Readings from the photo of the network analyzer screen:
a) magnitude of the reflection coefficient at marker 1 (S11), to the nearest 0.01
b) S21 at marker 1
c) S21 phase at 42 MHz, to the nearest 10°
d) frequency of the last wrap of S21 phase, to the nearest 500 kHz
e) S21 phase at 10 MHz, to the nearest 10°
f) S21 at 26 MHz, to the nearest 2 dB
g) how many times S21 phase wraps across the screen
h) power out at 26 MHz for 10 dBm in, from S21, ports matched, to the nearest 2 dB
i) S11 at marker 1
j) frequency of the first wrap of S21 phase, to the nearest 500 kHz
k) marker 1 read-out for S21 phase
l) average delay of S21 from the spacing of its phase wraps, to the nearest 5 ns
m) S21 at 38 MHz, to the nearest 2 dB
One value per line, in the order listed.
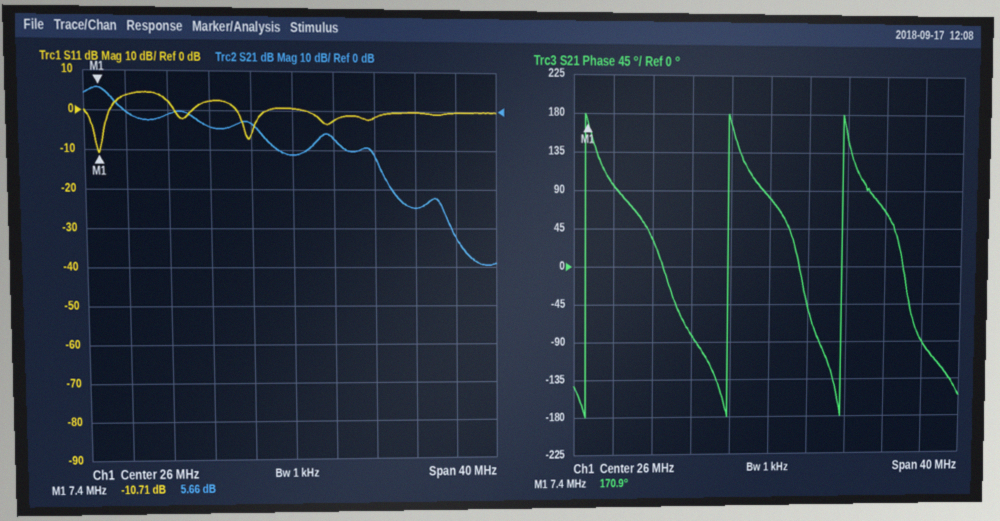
0.29
5.66 dB
-90°
33.5 MHz
100°
-12 dB
3
-2 dBm
-10.71 dB
7.0 MHz
170.9°
75 ns
-24 dB
